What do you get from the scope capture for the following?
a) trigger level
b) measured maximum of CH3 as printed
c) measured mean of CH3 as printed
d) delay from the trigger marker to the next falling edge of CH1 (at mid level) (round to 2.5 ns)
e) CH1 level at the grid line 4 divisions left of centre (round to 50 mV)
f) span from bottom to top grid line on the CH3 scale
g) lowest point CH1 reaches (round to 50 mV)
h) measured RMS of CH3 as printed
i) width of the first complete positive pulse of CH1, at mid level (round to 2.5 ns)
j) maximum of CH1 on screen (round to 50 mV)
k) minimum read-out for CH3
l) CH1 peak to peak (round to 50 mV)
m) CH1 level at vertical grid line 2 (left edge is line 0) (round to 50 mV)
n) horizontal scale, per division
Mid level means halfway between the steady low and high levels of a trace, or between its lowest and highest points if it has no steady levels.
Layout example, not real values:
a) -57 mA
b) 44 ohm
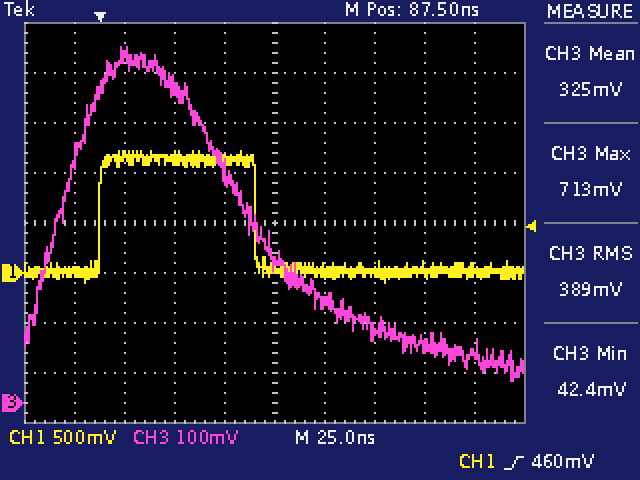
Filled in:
a) 460 mV
b) 713 mV
c) 325 mV
d) 77.5 ns
e) 0 mV
f) 800 mV
g) -100 mV
h) 389 mV
i) 77.5 ns
j) 1.20 V
k) 42.4 mV
l) 1.30 V
m) 1.15 V
n) 25 ns
